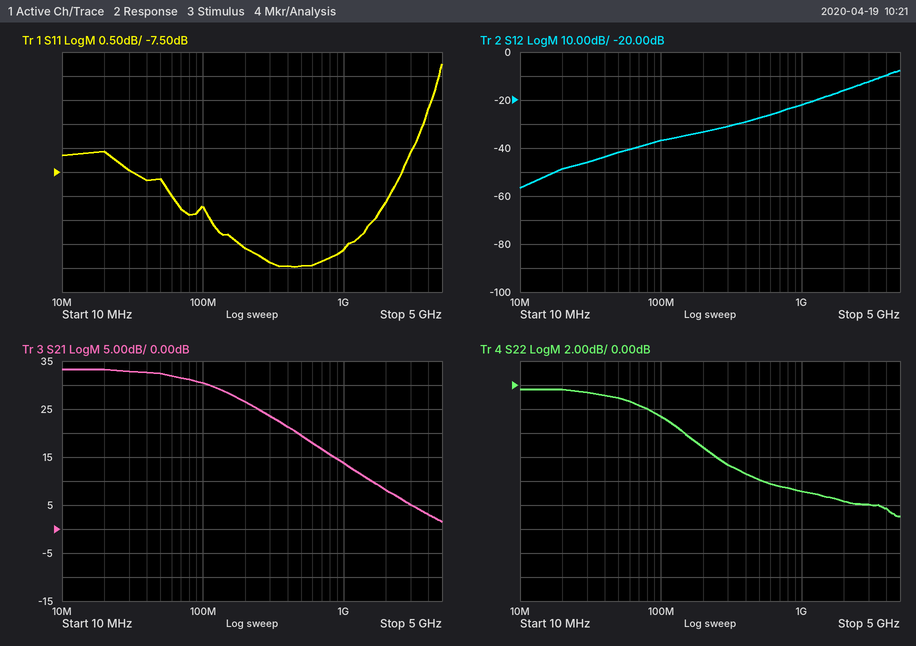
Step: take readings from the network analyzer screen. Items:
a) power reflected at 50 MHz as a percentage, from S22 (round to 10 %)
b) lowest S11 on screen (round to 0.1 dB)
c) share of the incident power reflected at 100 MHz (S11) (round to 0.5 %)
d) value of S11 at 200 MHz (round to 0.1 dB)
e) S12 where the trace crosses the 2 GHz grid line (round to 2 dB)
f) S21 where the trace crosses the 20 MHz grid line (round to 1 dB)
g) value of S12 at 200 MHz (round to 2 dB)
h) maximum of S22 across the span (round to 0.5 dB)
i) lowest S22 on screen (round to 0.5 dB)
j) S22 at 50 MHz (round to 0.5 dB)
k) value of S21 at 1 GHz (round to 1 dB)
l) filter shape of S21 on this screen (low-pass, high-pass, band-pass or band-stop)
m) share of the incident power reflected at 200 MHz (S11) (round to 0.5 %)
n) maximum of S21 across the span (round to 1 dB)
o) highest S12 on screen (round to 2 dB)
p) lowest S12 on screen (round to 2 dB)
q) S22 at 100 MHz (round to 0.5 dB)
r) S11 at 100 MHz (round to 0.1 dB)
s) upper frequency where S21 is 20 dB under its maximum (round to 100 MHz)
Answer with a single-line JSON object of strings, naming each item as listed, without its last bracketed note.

{"power reflected at 50 MHz as a percentage, from S22": "80 %", "lowest S11 on screen": "-9.5 dB", "share of the incident power reflected at 100 MHz (S11)": "15.0 %", "value of S11 at 200 MHz": "-9.1 dB", "S12 where the trace crosses the 2 GHz grid line": "-16 dB", "S21 where the trace crosses the 20 MHz grid line": "33 dB", "value of S12 at 200 MHz": "-34 dB", "maximum of S22 across the span": "-0.5 dB", "lowest S22 on screen": "-11.0 dB", "S22 at 50 MHz": "-1.0 dB", "value of S21 at 1 GHz": "14 dB", "filter shape of S21 on this screen": "low-pass", "share of the incident power reflected at 200 MHz (S11)": "12.5 %", "maximum of S21 across the span": "33 dB", "highest S12 on screen": "-8 dB", "lowest S12 on screen": "-56 dB", "S22 at 100 MHz": "-2.5 dB", "S11 at 100 MHz": "-8.2 dB", "upper frequency where S21 is 20 dB under its maximum": "1.1 GHz"}
